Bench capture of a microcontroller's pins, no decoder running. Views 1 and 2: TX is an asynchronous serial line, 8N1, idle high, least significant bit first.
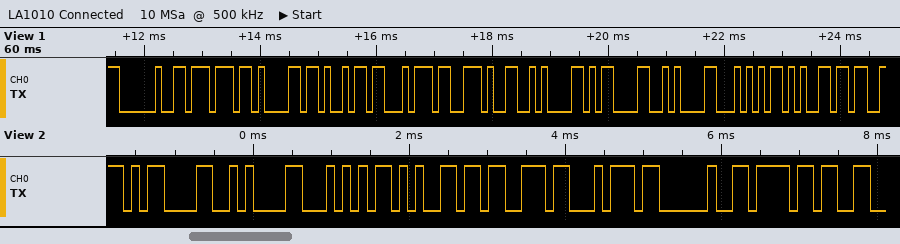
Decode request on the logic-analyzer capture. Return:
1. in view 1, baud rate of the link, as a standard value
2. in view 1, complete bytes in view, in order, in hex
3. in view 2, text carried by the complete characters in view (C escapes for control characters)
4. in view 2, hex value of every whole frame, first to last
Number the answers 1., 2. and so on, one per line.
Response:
1. 9600 baud
2. 0x20 0x77 0x61 0x69 0x74 0x2E 0x0A 0x0D 0x0A 0x54 0x65
3. "\r\nTest o"
4. 0D 0A 54 65 73 74 20 6F
